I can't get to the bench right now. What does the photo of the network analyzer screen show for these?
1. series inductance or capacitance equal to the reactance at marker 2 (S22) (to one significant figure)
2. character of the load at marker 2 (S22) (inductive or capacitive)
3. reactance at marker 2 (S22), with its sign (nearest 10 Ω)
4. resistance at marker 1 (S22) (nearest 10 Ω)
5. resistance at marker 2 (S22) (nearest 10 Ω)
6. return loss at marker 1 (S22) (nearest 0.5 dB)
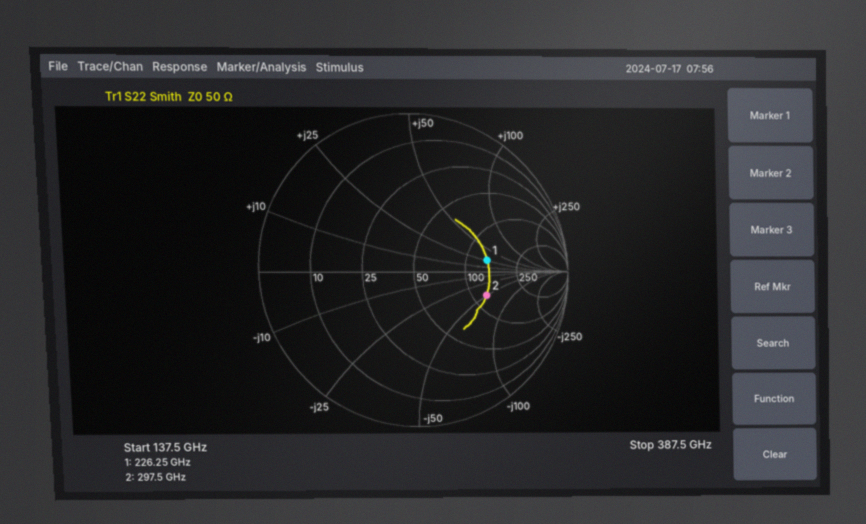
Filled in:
10 fF
capacitive
-50 Ω
140 Ω
120 Ω
6.5 dB
